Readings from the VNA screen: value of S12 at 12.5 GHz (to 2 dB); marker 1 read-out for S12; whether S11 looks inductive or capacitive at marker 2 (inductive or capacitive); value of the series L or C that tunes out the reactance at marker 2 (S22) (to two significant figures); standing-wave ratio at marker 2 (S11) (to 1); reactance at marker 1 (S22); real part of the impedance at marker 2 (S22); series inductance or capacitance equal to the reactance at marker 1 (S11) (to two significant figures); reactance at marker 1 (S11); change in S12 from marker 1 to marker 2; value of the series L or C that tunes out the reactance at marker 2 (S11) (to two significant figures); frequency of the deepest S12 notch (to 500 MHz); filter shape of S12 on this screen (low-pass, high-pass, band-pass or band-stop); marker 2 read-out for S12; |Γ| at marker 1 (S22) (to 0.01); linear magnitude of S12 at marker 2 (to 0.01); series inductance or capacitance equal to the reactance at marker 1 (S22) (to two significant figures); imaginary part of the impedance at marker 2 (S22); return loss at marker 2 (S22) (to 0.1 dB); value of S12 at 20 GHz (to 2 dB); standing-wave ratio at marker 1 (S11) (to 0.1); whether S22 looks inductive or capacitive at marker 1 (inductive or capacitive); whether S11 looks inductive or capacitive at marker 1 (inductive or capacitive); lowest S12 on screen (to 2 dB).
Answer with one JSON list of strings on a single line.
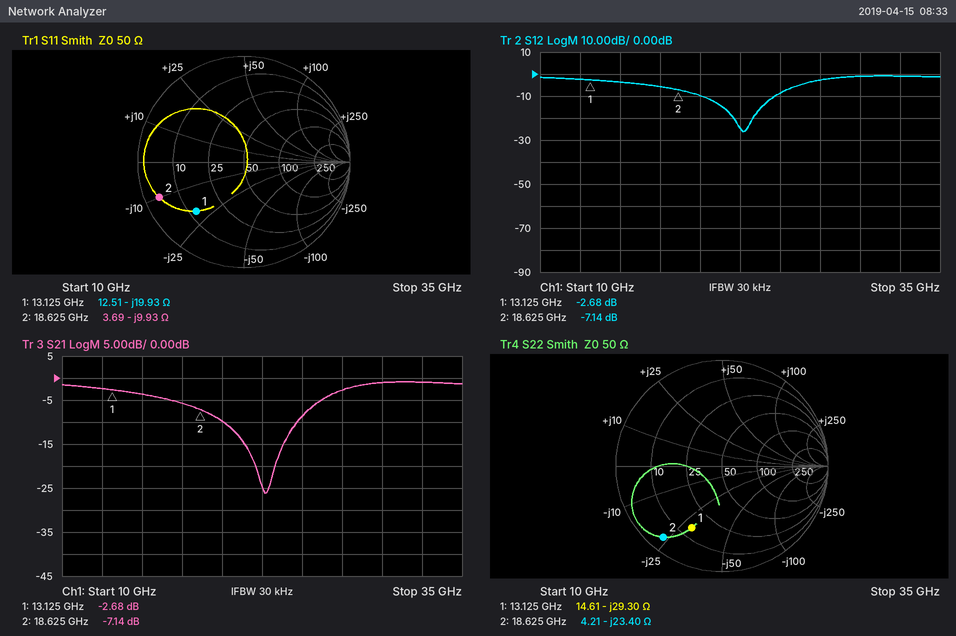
["-2 dB", "-2.68 dB", "capacitive", "200 pH", "14", "-29.30 Ω", "4.21 Ω", "610 fF", "-19.93 Ω", "-4.46 dB", "85 pH", "22.5 GHz", "band-stop", "-7.14 dB", "0.65", "0.44", "410 fF", "-23.40 Ω", "1.2 dB", "-10 dB", "4.7", "capacitive", "capacitive", "-26 dB"]
